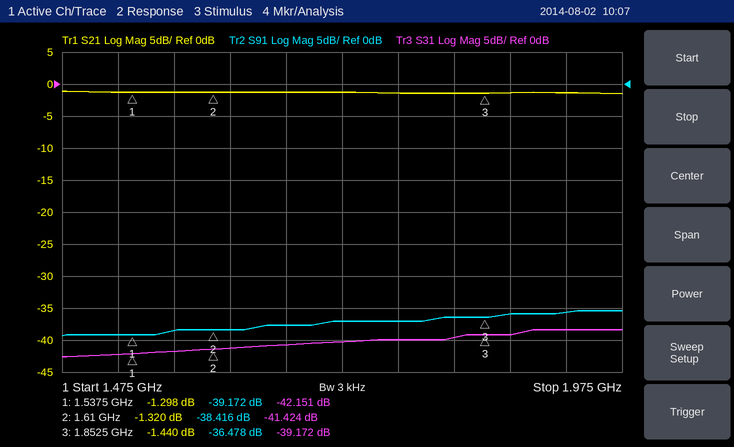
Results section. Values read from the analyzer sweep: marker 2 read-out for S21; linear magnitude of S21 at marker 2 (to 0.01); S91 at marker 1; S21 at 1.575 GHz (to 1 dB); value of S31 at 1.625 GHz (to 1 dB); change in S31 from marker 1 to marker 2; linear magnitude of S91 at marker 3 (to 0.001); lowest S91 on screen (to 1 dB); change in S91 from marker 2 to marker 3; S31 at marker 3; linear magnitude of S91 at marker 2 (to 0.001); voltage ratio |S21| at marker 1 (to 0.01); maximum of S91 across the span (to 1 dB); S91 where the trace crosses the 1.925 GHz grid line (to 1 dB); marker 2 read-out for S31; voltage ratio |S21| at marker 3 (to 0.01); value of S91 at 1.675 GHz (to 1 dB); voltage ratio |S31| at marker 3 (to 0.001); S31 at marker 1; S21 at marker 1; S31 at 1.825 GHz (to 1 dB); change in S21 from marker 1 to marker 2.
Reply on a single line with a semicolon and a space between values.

-1.320 dB; 0.86; -39.172 dB; -1 dB; -41 dB; 0.727 dB; 0.015; -39 dB; 1.938 dB; -39.172 dB; 0.012; 0.86; -35 dB; -36 dB; -41.424 dB; 0.85; -38 dB; 0.011; -42.151 dB; -1.298 dB; -40 dB; -0.022 dB
